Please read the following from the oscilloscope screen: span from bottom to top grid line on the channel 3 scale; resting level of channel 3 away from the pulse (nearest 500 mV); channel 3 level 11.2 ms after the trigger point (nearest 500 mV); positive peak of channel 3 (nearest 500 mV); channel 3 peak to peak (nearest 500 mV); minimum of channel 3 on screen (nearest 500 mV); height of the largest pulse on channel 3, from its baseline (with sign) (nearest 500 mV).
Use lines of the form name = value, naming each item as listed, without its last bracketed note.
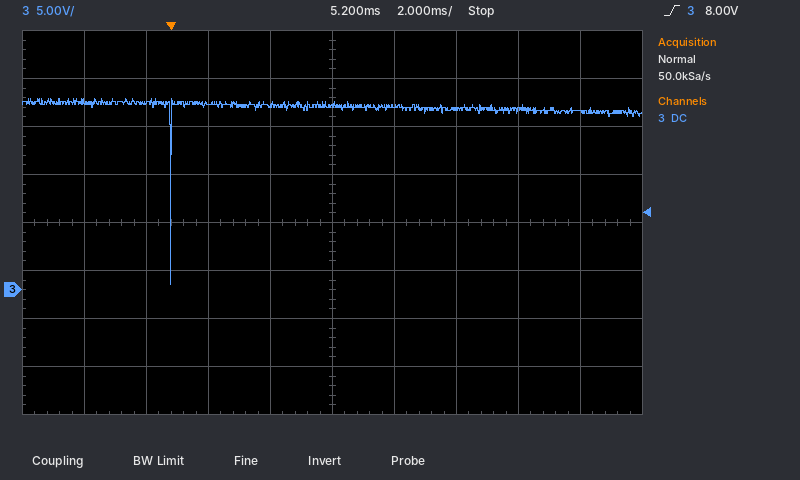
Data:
span from bottom to top grid line on the channel 3 scale = 40 V
resting level of channel 3 away from the pulse = 19.0 V
channel 3 level 11.2 ms after the trigger point = 18.5 V
positive peak of channel 3 = 20.0 V
channel 3 peak to peak = 19.5 V
minimum of channel 3 on screen = 500 mV
height of the largest pulse on channel 3, from its baseline (with sign) = -18.5 V
